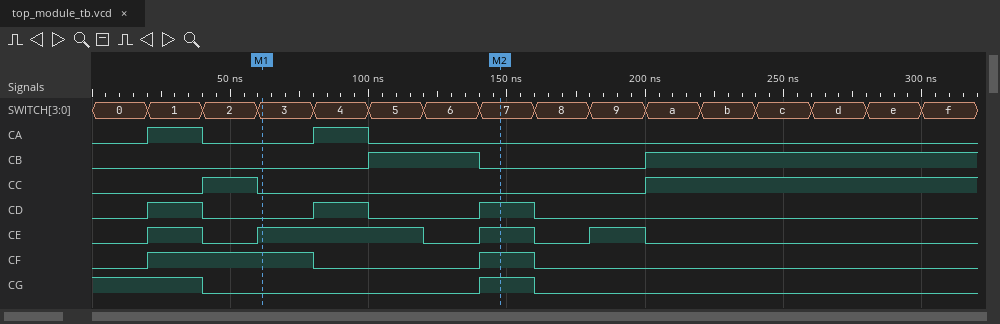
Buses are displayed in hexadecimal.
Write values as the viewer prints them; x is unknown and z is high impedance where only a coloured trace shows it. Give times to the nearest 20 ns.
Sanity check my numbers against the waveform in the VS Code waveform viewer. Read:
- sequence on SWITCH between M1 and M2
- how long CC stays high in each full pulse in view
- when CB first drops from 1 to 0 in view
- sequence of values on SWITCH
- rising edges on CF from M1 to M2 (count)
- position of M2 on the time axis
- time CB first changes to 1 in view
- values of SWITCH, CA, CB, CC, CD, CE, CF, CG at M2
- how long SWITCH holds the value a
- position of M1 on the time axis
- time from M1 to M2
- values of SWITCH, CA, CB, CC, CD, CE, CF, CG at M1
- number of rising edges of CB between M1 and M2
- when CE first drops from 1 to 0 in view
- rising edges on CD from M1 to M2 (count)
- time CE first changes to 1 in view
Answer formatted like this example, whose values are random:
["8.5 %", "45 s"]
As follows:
["3, 4, 5, 6, 7", "20 ns", "140 ns", "0, 1, 2, 3, 4, 5, 6, 7, 8, 9, a, b, c, d, e, f", "1", "140 ns", "100 ns", "SWITCH=7, CA=0, CB=0, CC=0, CD=1, CE=1, CF=1, CG=1", "20 ns", "60 ns", "80 ns", "SWITCH=3, CA=0, CB=0, CC=0, CD=0, CE=1, CF=1, CG=0", "1", "40 ns", "2", "20 ns"]
